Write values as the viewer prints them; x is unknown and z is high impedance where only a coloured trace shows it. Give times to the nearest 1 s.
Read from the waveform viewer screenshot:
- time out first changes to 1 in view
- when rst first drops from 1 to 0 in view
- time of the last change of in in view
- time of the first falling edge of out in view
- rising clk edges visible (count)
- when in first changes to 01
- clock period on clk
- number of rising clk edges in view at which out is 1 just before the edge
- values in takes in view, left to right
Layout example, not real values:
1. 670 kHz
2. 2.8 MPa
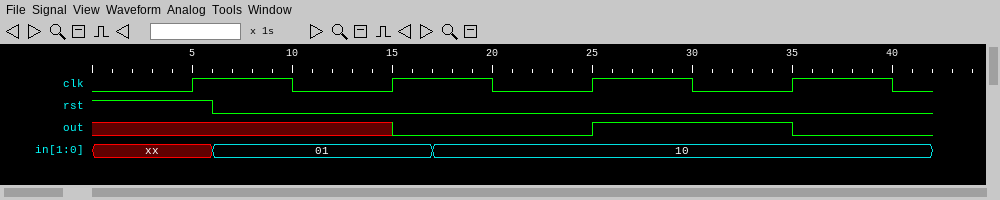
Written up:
1. 25 s
2. 6 s
3. 17 s
4. 35 s
5. 4
6. 6 s
7. 10 s
8. 1
9. xx, 01, 10
